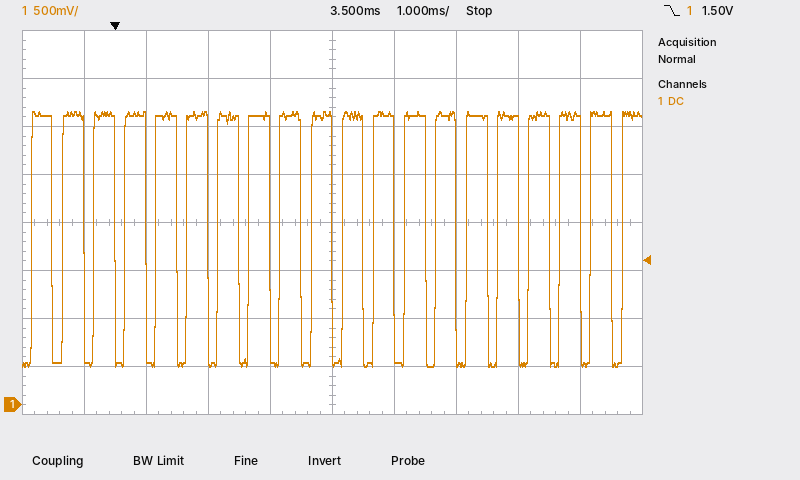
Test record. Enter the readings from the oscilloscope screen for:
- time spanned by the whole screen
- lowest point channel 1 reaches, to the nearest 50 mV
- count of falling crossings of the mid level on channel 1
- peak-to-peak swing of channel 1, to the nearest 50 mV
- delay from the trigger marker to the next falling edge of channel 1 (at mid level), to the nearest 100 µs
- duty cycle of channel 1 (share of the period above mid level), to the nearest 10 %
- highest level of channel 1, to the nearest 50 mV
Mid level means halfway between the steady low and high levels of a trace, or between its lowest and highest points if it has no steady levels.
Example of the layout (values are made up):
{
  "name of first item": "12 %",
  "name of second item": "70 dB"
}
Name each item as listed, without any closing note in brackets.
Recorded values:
{
  "time spanned by the whole screen": "10 ms",
  "lowest point channel 1 reaches, to the nearest 50 mV": "400 mV",
  "count of falling crossings of the mid level on channel 1": "19",
  "peak-to-peak swing of channel 1, to the nearest 50 mV": "2.65 V",
  "delay from the trigger marker to the next falling edge of channel 1 (at mid level), to the nearest 100 µs": "500 µs",
  "duty cycle of channel 1 (share of the period above mid level), to the nearest 10 %": "70 %",
  "highest level of channel 1, to the nearest 50 mV": "3.05 V"
}
